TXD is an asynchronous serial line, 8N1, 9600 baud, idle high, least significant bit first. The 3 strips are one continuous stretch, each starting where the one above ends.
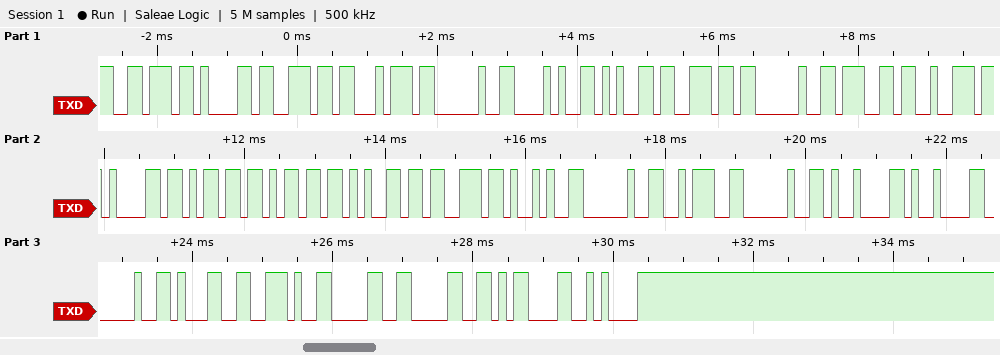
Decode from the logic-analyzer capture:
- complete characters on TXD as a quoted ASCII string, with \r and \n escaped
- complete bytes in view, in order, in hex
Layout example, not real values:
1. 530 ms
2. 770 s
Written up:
1. "vant (en grammes) : \t\t 1.00\r\n"
2. 76 61 6E 74 20 28 65 6E 20 67 72 61 6D 6D 65 73 29 20 3A 20 09 09 20 31 2E 30 30 0D 0A
